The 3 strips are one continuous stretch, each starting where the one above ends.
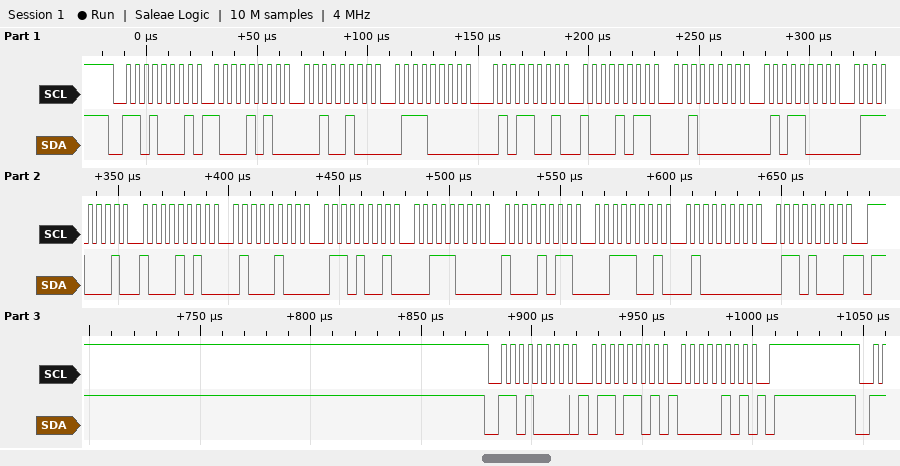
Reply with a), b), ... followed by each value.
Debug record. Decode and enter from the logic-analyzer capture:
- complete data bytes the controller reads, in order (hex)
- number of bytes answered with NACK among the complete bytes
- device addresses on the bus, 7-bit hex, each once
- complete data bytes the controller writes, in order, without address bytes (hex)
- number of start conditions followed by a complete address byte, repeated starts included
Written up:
a) 8A 24 70 59 8B 20 58 71 8A 44 69 38 8B 39 40 68
b) 1
c) 0x68
d) 6D 05
e) 2
